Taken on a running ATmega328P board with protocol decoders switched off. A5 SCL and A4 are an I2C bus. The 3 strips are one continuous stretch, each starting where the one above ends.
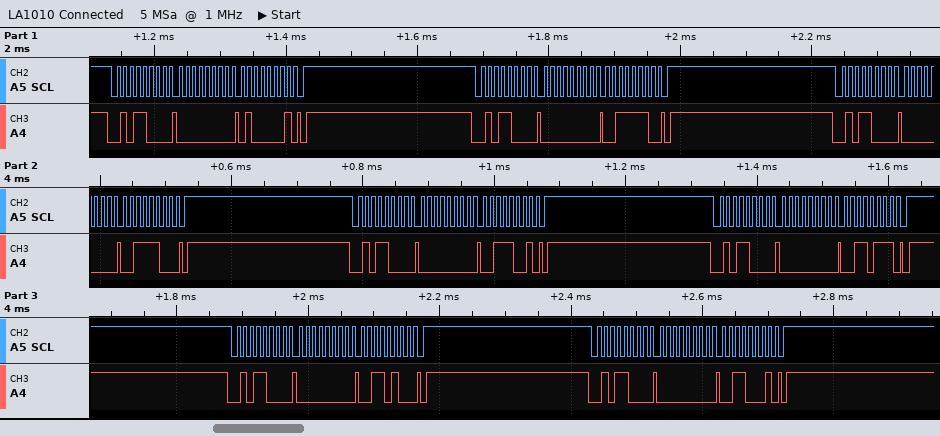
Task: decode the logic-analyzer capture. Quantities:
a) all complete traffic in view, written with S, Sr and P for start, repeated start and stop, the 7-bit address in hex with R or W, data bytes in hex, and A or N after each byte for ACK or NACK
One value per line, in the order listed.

S 2CW A 00 A 41 A P S 2CW A 00 A 3E A P S 2CW A 00 A 3C A P S 2CW A 00 A 39 A P S 2CW A 00 A 37 A P S 2CW A 00 A 34 A P S 2CW A 00 A 31 A P
